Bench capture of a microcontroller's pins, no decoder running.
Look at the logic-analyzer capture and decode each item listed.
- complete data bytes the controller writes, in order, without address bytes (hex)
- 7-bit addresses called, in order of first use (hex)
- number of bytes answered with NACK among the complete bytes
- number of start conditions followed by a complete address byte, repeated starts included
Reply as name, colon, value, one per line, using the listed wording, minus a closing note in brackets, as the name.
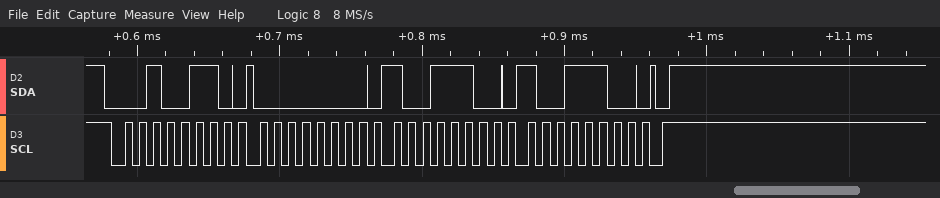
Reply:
complete data bytes the controller writes, in order, without address bytes: 00 9C 9C
7-bit addresses called, in order of first use: 0x13
number of bytes answered with NACK among the complete bytes: 0
number of start conditions followed by a complete address byte, repeated starts included: 1
